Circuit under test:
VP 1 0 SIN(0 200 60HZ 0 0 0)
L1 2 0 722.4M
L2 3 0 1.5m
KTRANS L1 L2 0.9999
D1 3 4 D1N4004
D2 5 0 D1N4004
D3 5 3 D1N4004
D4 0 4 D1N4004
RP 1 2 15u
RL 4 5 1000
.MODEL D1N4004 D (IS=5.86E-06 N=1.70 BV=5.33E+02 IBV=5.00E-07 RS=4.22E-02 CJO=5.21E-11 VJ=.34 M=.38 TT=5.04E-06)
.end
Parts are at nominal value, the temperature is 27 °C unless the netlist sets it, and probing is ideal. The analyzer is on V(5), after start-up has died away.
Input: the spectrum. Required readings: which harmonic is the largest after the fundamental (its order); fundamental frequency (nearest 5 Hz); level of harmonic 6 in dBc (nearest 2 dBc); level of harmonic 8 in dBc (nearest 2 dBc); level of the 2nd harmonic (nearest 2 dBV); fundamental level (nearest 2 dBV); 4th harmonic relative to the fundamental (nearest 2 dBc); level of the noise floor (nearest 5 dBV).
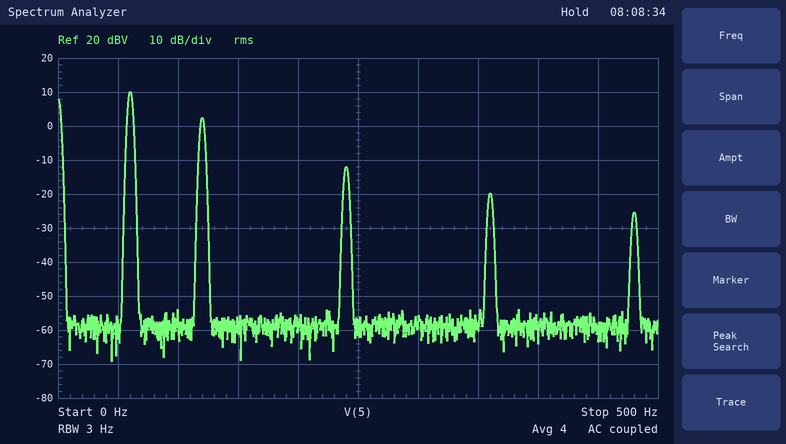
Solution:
2
60 Hz
-30 dBc
-36 dBc
2 dBV
10 dBV
-22 dBc
-60 dBV
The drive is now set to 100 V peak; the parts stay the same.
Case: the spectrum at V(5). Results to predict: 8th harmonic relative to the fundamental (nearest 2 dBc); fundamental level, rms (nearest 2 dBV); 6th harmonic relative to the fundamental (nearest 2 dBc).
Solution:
-38 dBc
4 dBV
-32 dBc
